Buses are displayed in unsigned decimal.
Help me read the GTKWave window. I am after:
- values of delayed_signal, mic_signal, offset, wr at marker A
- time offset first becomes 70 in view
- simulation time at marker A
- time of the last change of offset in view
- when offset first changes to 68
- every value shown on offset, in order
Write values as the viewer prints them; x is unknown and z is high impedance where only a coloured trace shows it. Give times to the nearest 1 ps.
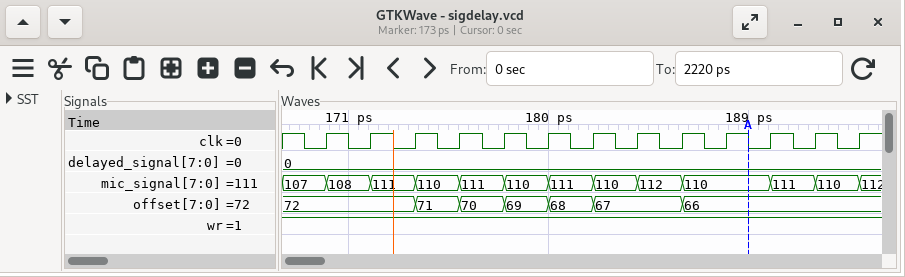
delayed_signal=0, mic_signal=110, offset=66, wr=1
176 ps
189 ps
186 ps
180 ps
72, 71, 70, 69, 68, 67, 66
